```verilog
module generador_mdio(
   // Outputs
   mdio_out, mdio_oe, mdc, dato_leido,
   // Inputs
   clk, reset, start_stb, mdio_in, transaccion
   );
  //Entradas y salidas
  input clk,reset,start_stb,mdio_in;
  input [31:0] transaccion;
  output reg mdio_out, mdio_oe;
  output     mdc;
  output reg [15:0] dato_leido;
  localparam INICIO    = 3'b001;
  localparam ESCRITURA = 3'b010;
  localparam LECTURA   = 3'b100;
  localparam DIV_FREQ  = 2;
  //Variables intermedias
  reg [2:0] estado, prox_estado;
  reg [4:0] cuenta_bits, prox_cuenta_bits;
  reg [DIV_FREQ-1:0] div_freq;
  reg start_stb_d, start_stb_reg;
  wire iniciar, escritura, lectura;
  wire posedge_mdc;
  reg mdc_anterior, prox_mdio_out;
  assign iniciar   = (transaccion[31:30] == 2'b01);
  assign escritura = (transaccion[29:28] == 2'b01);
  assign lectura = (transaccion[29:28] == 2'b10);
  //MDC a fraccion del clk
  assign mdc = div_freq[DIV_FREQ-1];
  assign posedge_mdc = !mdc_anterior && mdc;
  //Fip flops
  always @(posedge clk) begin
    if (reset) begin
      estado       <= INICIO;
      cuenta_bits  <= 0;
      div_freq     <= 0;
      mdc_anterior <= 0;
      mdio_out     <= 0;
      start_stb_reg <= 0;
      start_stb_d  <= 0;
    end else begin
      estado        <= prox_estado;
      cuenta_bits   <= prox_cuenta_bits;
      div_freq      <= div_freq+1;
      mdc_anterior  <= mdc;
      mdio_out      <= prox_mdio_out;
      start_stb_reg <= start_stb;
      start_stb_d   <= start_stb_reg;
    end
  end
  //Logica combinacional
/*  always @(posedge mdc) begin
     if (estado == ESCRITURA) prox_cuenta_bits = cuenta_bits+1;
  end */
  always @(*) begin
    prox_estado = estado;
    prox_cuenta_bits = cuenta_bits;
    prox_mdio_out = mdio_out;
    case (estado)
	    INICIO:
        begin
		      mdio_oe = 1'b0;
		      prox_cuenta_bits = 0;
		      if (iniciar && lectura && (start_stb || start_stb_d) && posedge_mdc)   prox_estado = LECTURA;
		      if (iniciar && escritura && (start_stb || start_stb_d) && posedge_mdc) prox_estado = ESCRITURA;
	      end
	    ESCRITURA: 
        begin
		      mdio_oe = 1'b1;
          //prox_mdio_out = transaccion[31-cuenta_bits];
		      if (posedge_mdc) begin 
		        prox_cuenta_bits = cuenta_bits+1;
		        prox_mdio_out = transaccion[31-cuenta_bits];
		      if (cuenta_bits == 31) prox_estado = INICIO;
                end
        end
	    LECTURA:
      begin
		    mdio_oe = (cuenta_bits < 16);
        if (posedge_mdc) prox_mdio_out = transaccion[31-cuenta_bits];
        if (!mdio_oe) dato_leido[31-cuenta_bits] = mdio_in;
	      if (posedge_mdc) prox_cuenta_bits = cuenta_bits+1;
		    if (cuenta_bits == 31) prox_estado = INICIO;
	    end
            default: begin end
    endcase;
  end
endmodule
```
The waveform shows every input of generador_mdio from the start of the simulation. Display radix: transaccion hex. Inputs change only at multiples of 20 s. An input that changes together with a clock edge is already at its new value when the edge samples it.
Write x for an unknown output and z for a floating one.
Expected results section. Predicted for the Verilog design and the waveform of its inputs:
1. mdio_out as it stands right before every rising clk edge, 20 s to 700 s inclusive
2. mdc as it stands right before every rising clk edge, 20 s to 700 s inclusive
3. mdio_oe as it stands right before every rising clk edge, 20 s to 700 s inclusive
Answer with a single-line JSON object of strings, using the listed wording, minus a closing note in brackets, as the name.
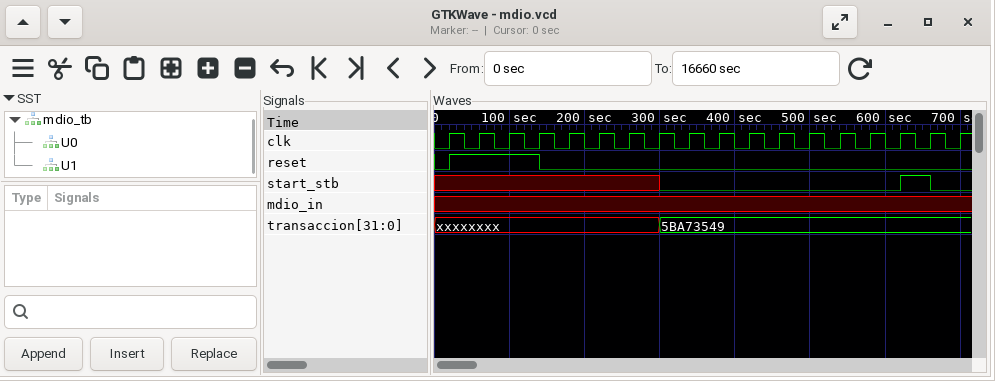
{"mdio_out as it stands right before every rising clk edge, 20 s to 700 s inclusive": "x 0 0 0 0 0 0 0 0 0 0 0 0 0 0 0 0 0", "mdc as it stands right before every rising clk edge, 20 s to 700 s inclusive": "x 0 0 0 0 1 1 0 0 1 1 0 0 1 1 0 0 1", "mdio_oe as it stands right before every rising clk edge, 20 s to 700 s inclusive": "x 0 0 0 0 0 0 0 0 0 0 0 0 0 0 0 0 0"}
